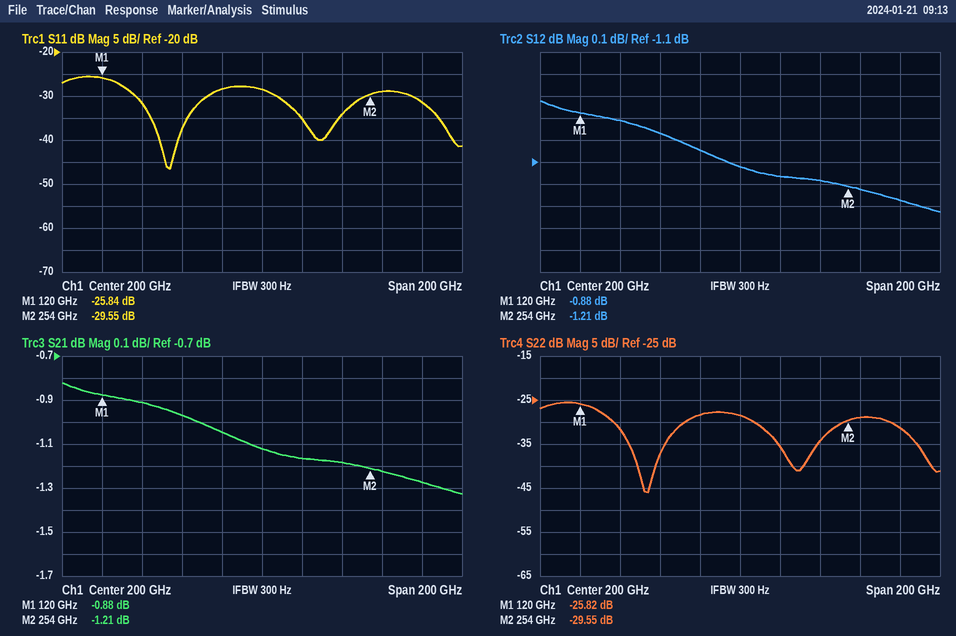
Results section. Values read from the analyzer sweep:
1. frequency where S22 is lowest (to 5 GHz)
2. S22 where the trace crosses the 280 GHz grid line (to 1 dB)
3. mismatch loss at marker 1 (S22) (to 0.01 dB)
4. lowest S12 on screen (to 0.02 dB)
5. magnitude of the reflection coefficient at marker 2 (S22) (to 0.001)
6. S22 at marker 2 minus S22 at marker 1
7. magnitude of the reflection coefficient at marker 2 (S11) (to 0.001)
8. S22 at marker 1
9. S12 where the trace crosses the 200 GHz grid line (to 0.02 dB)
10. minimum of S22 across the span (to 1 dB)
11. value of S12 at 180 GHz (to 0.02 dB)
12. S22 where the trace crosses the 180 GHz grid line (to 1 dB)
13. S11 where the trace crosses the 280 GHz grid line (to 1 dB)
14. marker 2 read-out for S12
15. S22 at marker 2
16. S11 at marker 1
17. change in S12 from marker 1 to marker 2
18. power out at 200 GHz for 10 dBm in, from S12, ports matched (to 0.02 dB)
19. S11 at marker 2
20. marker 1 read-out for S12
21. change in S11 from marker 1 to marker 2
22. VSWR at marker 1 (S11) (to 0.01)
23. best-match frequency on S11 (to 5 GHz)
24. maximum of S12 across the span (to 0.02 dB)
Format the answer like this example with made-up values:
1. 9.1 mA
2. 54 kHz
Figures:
1. 155 GHz
2. -31 dB
3. 0.01 dB
4. -1.32 dB
5. 0.033
6. -3.73 dB
7. 0.033
8. -25.82 dB
9. -1.12 dB
10. -46 dB
11. -1.04 dB
12. -28 dB
13. -31 dB
14. -1.21 dB
15. -29.55 dB
16. -25.84 dB
17. -0.33 dB
18. 8.88 dBm
19. -29.55 dB
20. -0.88 dB
21. -3.71 dB
22. 1.11
23. 155 GHz
24. -0.82 dB
